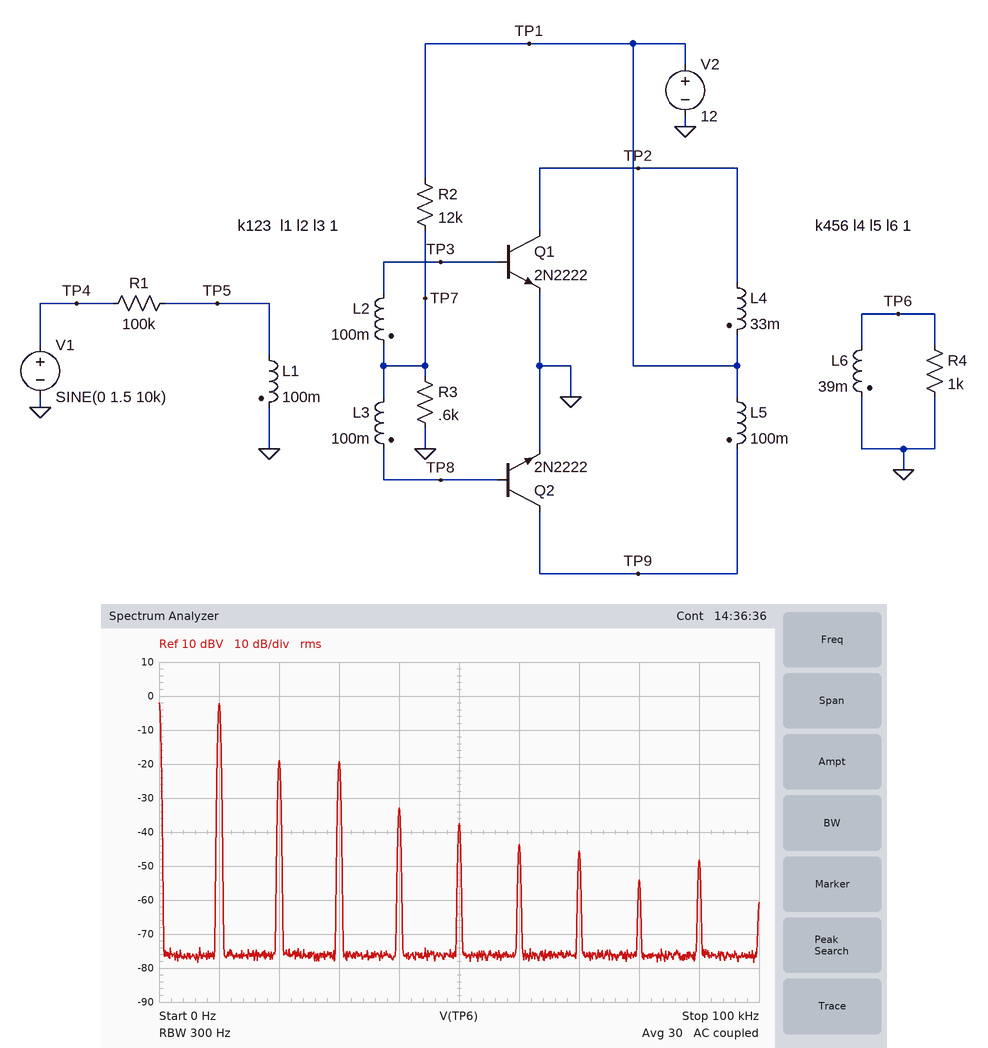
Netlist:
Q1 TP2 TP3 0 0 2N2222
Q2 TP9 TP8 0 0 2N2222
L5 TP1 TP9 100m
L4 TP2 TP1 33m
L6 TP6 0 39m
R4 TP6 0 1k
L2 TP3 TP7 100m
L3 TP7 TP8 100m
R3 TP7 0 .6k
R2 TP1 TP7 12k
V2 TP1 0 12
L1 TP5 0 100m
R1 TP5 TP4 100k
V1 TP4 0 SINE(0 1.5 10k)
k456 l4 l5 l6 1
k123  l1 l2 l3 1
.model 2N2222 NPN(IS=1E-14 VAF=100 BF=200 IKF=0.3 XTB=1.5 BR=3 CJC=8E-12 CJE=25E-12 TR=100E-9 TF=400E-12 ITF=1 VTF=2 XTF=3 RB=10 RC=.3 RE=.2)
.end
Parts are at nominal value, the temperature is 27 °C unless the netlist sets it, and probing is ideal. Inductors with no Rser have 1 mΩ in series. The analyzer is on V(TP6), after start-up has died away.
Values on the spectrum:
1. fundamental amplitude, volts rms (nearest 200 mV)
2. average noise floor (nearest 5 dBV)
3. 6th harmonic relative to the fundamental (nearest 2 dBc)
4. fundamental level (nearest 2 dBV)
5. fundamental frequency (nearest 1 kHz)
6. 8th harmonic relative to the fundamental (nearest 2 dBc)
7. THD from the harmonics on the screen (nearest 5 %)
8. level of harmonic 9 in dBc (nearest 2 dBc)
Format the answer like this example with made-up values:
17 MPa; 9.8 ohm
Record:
800 mV; -75 dBV; -42 dBc; -2 dBV; 10 kHz; -52 dBc; 20 %; -46 dBc
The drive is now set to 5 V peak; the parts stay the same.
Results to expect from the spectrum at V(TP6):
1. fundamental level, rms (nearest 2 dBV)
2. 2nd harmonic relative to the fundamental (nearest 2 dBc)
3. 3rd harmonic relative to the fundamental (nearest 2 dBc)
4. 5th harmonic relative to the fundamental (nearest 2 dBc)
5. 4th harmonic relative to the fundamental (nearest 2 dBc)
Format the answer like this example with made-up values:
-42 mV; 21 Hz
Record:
16 dBV; -20 dBc; -18 dBc; -38 dBc; -24 dBc
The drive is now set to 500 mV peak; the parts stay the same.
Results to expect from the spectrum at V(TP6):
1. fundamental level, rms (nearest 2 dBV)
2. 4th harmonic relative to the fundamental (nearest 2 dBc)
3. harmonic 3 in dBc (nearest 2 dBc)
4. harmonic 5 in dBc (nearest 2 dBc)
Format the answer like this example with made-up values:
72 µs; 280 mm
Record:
-20 dBV; -46 dBc; -24 dBc; -54 dBc
